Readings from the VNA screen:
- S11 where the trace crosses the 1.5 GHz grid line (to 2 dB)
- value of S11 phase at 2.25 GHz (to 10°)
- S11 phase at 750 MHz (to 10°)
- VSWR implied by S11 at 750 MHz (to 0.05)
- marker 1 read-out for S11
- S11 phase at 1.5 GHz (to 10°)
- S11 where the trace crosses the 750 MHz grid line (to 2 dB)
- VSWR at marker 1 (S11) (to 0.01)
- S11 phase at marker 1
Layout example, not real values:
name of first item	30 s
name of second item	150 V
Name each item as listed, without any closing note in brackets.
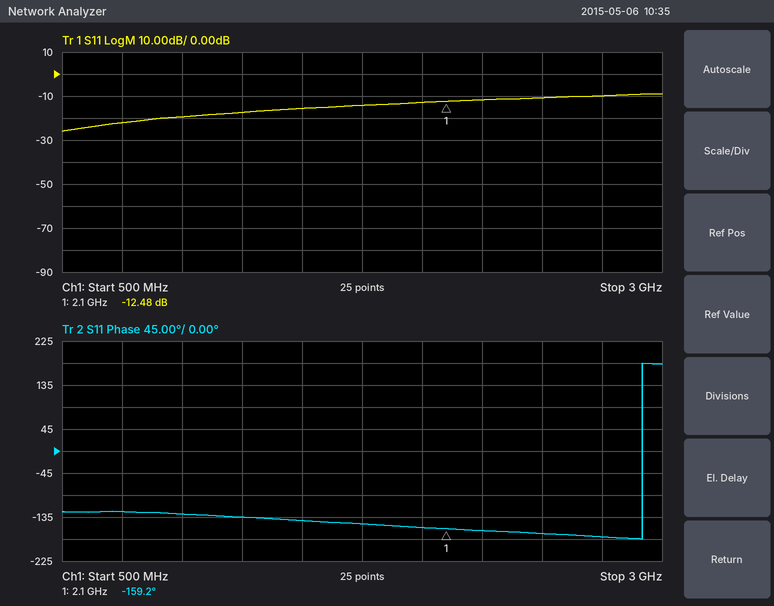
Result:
S11 where the trace crosses the 1.5 GHz grid line	-16 dB
value of S11 phase at 2.25 GHz	-160°
S11 phase at 750 MHz	-120°
VSWR implied by S11 at 750 MHz	1.15
marker 1 read-out for S11	-12.48 dB
S11 phase at 1.5 GHz	-140°
S11 where the trace crosses the 750 MHz grid line	-22 dB
VSWR at marker 1 (S11)	1.62
S11 phase at marker 1	-159.2°
